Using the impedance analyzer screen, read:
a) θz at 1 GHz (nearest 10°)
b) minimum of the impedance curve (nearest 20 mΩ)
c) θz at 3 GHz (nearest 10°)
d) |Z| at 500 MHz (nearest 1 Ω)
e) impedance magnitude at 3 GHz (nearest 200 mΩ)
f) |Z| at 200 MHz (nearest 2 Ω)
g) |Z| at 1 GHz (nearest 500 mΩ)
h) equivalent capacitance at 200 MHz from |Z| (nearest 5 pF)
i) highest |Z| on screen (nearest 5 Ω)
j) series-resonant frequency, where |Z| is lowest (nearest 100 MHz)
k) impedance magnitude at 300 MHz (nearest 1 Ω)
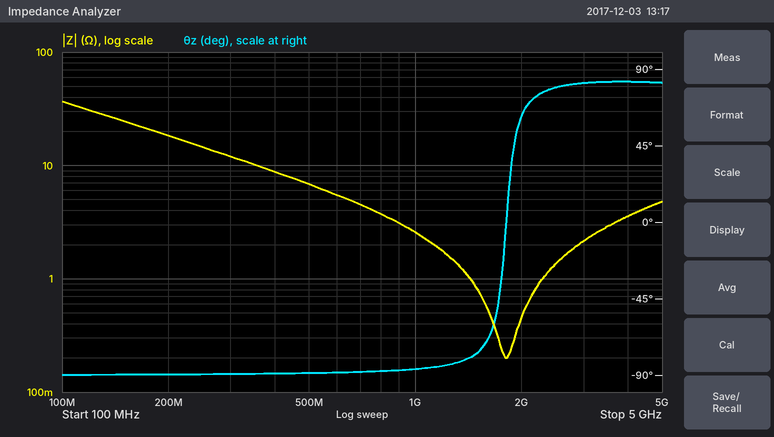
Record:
-90°
200 mΩ
80°
7 Ω
2.2 Ω
18 Ω
2.5 Ω
45 pF
35 Ω
1.8 GHz
12 Ω
